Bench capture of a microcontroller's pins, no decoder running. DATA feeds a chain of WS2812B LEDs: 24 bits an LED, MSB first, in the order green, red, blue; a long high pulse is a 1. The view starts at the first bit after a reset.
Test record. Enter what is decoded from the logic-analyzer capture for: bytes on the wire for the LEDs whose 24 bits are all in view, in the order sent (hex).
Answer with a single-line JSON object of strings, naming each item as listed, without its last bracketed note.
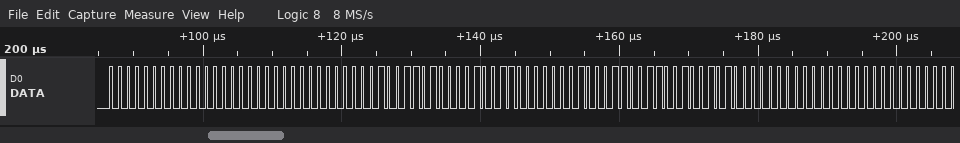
{"bytes on the wire for the LEDs whose 24 bits are all in view, in the order sent": "00 00 00 01 34 26 02 33 25 00 00 00"}
